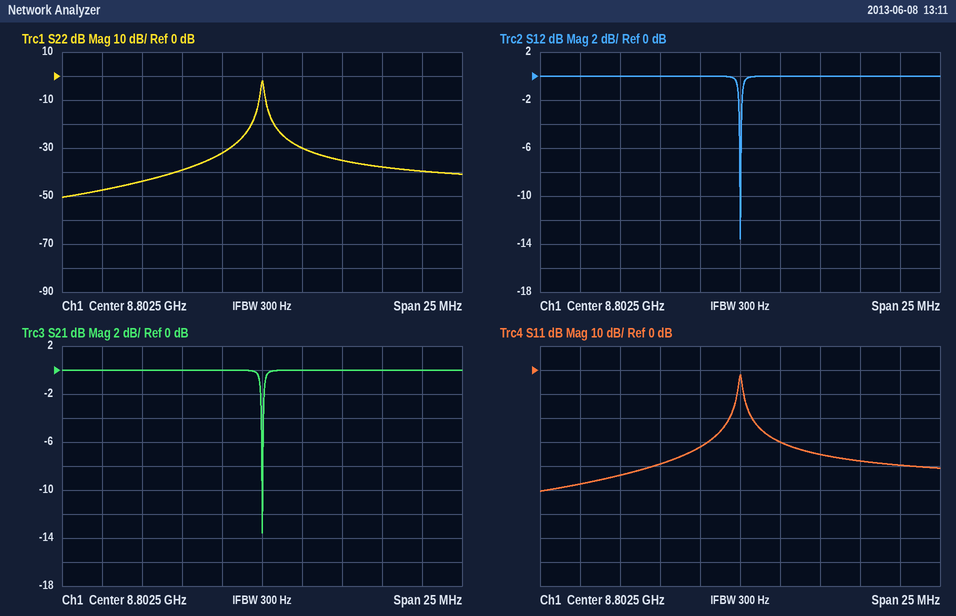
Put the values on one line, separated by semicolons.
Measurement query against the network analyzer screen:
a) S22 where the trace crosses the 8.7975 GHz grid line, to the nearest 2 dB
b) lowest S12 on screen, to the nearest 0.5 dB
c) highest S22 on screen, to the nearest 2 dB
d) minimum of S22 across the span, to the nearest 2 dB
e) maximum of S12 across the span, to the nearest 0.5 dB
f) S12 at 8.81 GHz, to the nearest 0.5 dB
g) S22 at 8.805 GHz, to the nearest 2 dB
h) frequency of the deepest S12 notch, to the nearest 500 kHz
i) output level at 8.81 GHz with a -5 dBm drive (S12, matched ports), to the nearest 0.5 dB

-40 dB; -13.5 dB; -2 dB; -50 dB; 0.0 dB; 0.0 dB; -30 dB; 8.8025 GHz; -5.0 dBm
